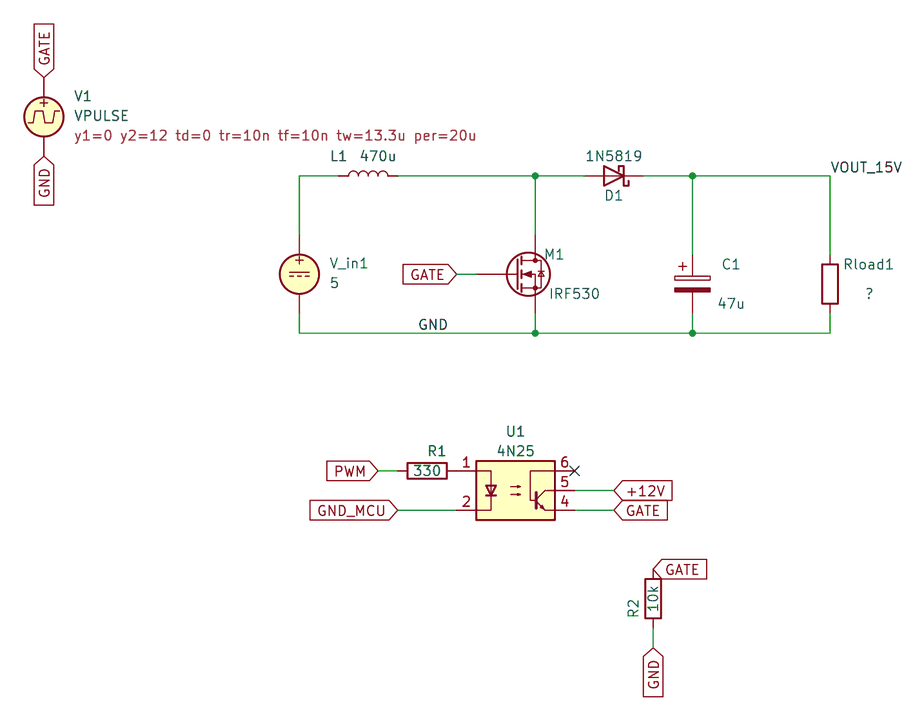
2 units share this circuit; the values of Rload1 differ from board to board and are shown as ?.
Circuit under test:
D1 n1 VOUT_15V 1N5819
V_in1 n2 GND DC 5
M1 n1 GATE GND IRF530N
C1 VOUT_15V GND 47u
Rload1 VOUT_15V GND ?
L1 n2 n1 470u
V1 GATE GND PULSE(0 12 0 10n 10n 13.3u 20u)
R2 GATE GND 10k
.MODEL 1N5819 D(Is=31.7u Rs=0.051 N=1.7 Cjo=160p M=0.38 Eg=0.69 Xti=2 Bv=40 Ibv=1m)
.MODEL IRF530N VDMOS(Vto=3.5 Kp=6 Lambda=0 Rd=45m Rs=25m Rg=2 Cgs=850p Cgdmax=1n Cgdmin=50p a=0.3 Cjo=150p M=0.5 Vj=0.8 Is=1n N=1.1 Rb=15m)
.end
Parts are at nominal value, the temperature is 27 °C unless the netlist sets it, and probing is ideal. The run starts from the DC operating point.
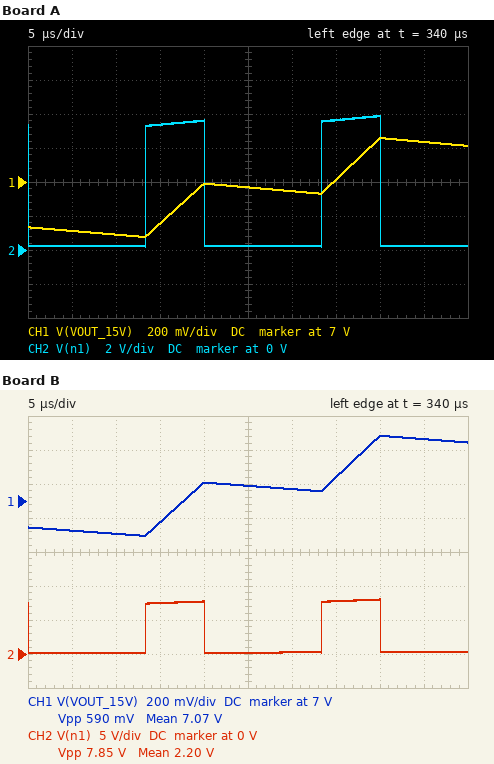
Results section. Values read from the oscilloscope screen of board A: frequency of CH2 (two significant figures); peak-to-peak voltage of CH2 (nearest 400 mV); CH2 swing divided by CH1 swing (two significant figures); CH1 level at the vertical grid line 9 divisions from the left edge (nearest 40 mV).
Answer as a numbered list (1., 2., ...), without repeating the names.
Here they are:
1. 50 kHz
2. 7.6 V
3. 13
4. 7.24 V
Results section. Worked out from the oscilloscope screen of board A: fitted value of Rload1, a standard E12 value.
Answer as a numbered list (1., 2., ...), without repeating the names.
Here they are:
1. 33 Ω
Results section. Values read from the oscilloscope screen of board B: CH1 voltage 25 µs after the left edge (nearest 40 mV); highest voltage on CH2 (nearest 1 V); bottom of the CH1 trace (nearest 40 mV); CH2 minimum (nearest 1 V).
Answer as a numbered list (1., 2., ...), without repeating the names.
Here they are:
1. 7.08 V
2. 8 V
3. 6.80 V
4. 0 V
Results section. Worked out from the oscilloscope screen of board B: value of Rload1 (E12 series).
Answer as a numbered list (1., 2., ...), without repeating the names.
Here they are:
1. 39 Ω
